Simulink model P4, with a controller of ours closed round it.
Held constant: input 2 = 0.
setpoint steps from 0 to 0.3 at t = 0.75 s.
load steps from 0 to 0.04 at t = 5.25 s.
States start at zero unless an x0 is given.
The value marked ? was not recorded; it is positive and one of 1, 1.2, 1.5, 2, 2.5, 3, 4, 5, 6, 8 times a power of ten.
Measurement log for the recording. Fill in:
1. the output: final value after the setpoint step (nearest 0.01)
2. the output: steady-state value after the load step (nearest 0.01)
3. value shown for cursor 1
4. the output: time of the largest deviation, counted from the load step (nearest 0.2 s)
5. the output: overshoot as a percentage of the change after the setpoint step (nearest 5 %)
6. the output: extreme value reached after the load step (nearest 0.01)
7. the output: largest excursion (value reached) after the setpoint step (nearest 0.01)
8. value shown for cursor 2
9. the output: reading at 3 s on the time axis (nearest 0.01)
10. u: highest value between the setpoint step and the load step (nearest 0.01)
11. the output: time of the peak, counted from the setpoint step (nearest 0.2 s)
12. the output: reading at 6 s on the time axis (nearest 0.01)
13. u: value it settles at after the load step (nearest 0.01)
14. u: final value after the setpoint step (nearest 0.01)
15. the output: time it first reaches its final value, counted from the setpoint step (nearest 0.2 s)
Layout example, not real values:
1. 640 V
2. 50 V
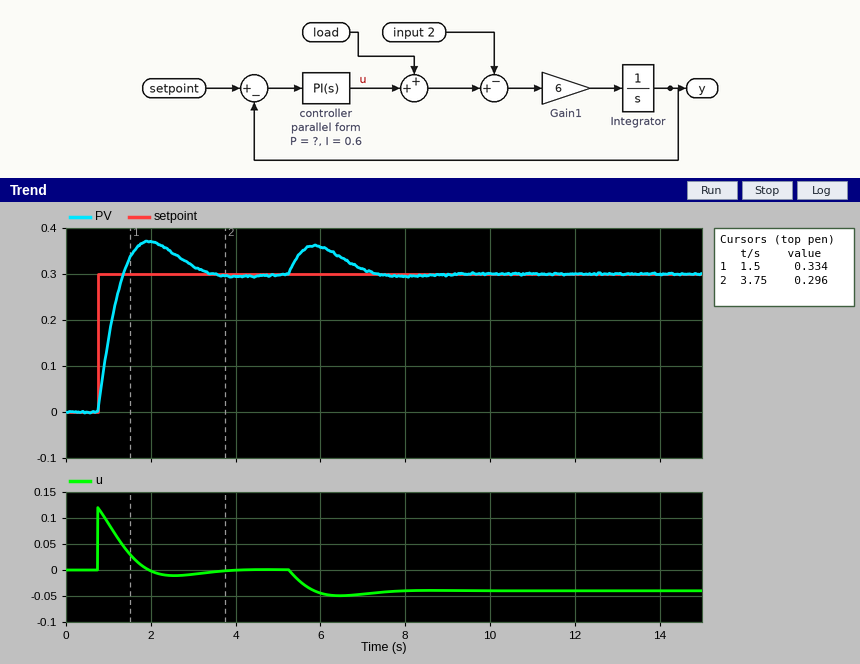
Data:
1. 0.30
2. 0.30
3. 0.334
4. 0.6 s
5. 25 %
6. 0.36
7. 0.37
8. 0.296
9. 0.32
10. 0.12
11. 1.2 s
12. 0.36
13. -0.04
14. 0.00
15. 0.6 s
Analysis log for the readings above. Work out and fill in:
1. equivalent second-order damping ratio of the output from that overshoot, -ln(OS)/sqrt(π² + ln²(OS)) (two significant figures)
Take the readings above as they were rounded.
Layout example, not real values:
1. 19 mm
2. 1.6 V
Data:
1. 0.40
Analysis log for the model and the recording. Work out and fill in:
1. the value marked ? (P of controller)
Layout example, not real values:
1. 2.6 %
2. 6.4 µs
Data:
1. 0.4
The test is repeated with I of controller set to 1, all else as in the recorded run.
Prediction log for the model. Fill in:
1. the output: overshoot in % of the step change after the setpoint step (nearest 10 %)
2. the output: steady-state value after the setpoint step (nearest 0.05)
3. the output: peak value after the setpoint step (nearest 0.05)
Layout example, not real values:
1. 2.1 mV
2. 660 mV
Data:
1. 30 %
2. 0.30
3. 0.40
